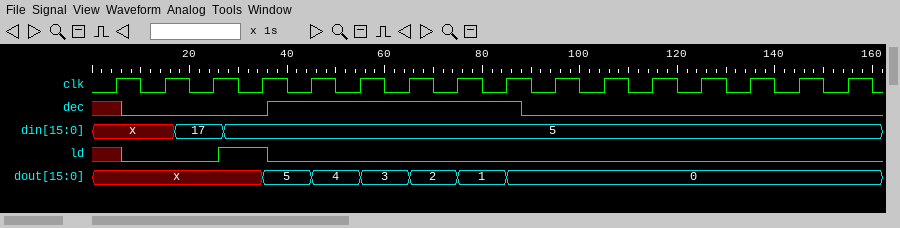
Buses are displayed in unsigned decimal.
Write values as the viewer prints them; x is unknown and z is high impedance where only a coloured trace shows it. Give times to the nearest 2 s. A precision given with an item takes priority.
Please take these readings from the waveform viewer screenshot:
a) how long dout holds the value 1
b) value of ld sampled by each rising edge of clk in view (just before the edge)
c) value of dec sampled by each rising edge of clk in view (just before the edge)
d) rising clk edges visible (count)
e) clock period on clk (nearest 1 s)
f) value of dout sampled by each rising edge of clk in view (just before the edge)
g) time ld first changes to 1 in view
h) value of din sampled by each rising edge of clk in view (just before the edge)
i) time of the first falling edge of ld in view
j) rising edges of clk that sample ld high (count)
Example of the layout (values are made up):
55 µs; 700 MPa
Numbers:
10 s; x 0 0 1 0 0 0 0 0 0 0 0 0 0 0 0; x 0 0 0 1 1 1 1 1 0 0 0 0 0 0 0; 16; 10 s; x, x, x, x, 5, 4, 3, 2, 1, 0, 0, 0, 0, 0, 0, 0; 26 s; x, x, 17, 5, 5, 5, 5, 5, 5, 5, 5, 5, 5, 5, 5, 5; 36 s; 1
